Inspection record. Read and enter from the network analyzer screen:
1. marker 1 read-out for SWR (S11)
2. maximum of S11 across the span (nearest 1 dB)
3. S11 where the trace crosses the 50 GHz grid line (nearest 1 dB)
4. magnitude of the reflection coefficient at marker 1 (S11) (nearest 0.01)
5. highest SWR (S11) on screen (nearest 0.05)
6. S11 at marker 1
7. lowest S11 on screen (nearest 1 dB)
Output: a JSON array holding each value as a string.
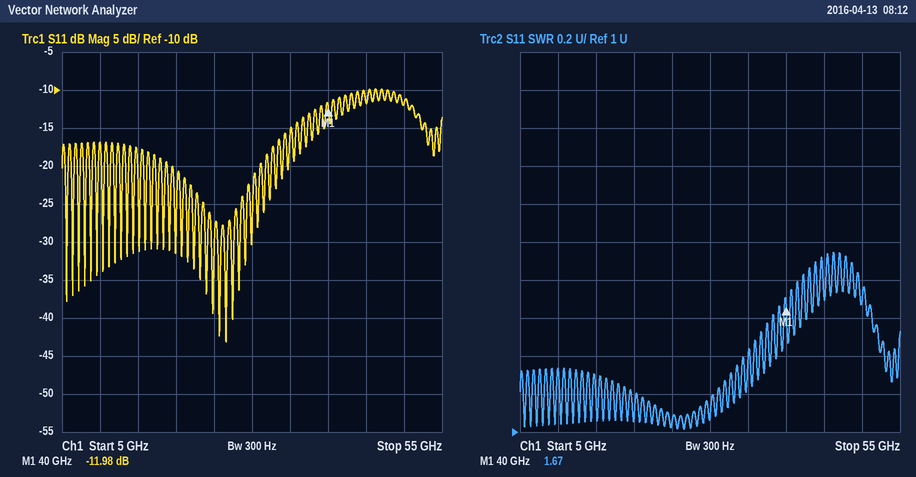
["1.67", "-10 dB", "-12 dB", "0.25", "1.95", "-11.98 dB", "-43 dB"]
